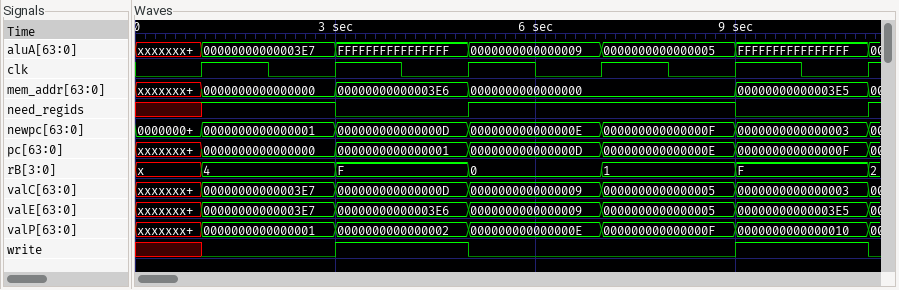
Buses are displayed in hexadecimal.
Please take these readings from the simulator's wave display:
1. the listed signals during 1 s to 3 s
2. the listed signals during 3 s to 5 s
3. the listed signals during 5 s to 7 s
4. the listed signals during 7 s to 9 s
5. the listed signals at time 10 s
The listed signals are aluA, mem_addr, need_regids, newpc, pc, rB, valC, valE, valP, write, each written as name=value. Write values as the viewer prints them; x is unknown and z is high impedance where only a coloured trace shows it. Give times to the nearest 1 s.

aluA=00000000000003E7, mem_addr=0000000000000000, need_regids=1, newpc=0000000000000001, pc=0000000000000000, rB=4, valC=00000000000003E7, valE=00000000000003E7, valP=0000000000000001, write=0
aluA=FFFFFFFFFFFFFFFF, mem_addr=00000000000003E6, need_regids=0, newpc=000000000000000D, pc=0000000000000001, rB=F, valC=000000000000000D, valE=00000000000003E6, valP=0000000000000002, write=1
aluA=0000000000000009, mem_addr=0000000000000000, need_regids=1, newpc=000000000000000E, pc=000000000000000D, rB=0, valC=0000000000000009, valE=0000000000000009, valP=000000000000000E, write=0
aluA=0000000000000005, mem_addr=0000000000000000, need_regids=1, newpc=000000000000000F, pc=000000000000000E, rB=1, valC=0000000000000005, valE=0000000000000005, valP=000000000000000F, write=0
aluA=FFFFFFFFFFFFFFFF, mem_addr=00000000000003E5, need_regids=0, newpc=0000000000000003, pc=000000000000000F, rB=F, valC=0000000000000003, valE=00000000000003E5, valP=0000000000000010, write=1
